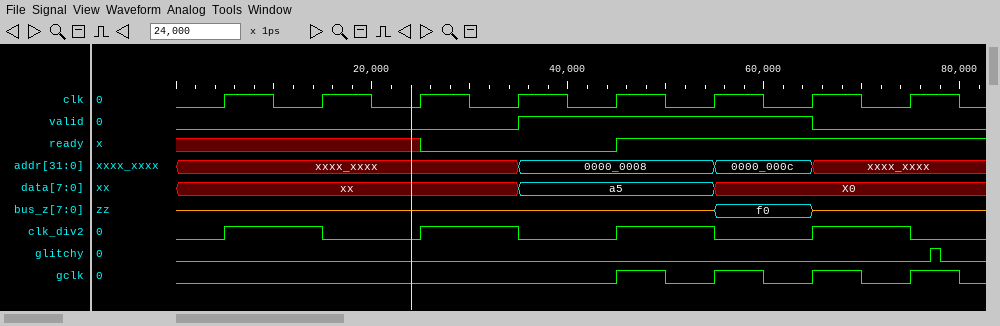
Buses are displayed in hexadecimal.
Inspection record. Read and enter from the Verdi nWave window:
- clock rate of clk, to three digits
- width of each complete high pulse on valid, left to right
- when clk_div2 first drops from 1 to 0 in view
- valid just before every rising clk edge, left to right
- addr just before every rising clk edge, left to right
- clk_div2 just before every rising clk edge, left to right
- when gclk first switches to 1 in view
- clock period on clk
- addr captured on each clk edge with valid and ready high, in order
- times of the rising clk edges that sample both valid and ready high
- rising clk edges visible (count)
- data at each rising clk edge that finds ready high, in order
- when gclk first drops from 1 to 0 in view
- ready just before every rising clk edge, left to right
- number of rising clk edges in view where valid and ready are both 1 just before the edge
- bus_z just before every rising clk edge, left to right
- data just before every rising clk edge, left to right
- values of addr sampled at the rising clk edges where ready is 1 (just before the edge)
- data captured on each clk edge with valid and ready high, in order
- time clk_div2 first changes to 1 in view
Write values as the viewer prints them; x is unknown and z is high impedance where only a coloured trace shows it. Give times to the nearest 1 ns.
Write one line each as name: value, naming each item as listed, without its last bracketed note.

clock rate of clk, to three digits: 100 MHz
width of each complete high pulse on valid, left to right: 30 ns
when clk_div2 first drops from 1 to 0 in view: 15 ns
valid just before every rising clk edge, left to right: 0 0 0 0 1 1 1 0
addr just before every rising clk edge, left to right: xxxx_xxxx, xxxx_xxxx, xxxx_xxxx, xxxx_xxxx, 0000_0008, 0000_0008, 0000_000c, xxxx_xxxx
clk_div2 just before every rising clk edge, left to right: 0 1 0 1 0 1 0 1
when gclk first switches to 1 in view: 45 ns
clock period on clk: 10 ns
addr captured on each clk edge with valid and ready high, in order: 0000_0008, 0000_000c
times of the rising clk edges that sample both valid and ready high: 55 ns, 65 ns
rising clk edges visible: 8
data at each rising clk edge that finds ready high, in order: a5, X0, X0
when gclk first drops from 1 to 0 in view: 50 ns
ready just before every rising clk edge, left to right: x x x 0 0 1 1 1
number of rising clk edges in view where valid and ready are both 1 just before the edge: 2
bus_z just before every rising clk edge, left to right: z, z, z, z, z, z, f0, z
data just before every rising clk edge, left to right: xx, xx, xx, xx, a5, a5, X0, X0
values of addr sampled at the rising clk edges where ready is 1: 0000_0008, 0000_000c, xxxx_xxxx
data captured on each clk edge with valid and ready high, in order: a5, X0
time clk_div2 first changes to 1 in view: 5 ns
